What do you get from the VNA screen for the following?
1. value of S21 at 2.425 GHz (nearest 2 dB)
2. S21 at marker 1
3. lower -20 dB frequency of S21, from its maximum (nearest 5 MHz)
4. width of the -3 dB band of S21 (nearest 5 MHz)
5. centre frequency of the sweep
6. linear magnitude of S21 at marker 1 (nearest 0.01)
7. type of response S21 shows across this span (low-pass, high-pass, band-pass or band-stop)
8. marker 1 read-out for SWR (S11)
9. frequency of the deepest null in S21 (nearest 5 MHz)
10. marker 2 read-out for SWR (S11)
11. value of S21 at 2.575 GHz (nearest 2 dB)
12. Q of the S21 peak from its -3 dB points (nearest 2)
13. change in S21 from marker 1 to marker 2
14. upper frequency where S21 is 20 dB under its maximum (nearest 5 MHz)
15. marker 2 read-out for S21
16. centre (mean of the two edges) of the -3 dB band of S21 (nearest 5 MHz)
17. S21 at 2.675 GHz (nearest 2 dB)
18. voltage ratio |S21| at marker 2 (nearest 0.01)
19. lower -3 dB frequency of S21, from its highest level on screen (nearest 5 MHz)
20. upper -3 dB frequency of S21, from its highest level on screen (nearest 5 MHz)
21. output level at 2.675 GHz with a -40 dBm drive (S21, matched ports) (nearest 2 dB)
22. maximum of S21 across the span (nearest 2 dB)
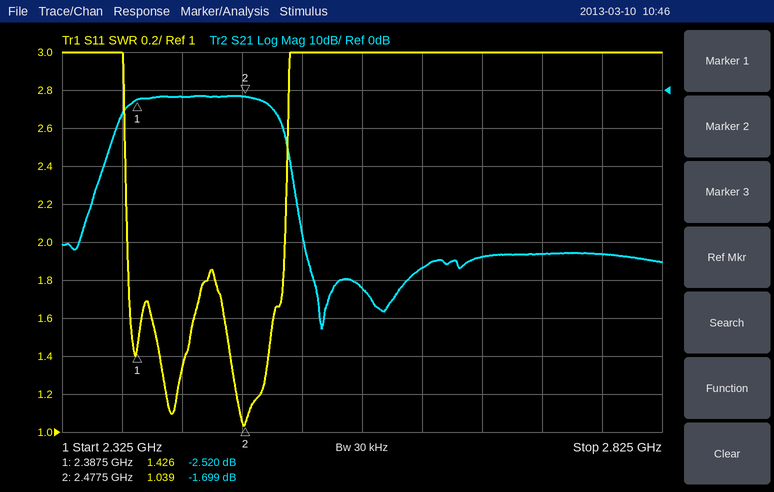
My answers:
-2 dB
-2.520 dB
2.360 GHz
120 MHz
2.575 GHz
0.75
band-pass
1.426
2.540 GHz
1.039
-52 dB
20
0.821 dB
2.515 GHz
-1.699 dB
2.440 GHz
-44 dB
0.82
2.380 GHz
2.500 GHz
-84 dBm
-2 dB
